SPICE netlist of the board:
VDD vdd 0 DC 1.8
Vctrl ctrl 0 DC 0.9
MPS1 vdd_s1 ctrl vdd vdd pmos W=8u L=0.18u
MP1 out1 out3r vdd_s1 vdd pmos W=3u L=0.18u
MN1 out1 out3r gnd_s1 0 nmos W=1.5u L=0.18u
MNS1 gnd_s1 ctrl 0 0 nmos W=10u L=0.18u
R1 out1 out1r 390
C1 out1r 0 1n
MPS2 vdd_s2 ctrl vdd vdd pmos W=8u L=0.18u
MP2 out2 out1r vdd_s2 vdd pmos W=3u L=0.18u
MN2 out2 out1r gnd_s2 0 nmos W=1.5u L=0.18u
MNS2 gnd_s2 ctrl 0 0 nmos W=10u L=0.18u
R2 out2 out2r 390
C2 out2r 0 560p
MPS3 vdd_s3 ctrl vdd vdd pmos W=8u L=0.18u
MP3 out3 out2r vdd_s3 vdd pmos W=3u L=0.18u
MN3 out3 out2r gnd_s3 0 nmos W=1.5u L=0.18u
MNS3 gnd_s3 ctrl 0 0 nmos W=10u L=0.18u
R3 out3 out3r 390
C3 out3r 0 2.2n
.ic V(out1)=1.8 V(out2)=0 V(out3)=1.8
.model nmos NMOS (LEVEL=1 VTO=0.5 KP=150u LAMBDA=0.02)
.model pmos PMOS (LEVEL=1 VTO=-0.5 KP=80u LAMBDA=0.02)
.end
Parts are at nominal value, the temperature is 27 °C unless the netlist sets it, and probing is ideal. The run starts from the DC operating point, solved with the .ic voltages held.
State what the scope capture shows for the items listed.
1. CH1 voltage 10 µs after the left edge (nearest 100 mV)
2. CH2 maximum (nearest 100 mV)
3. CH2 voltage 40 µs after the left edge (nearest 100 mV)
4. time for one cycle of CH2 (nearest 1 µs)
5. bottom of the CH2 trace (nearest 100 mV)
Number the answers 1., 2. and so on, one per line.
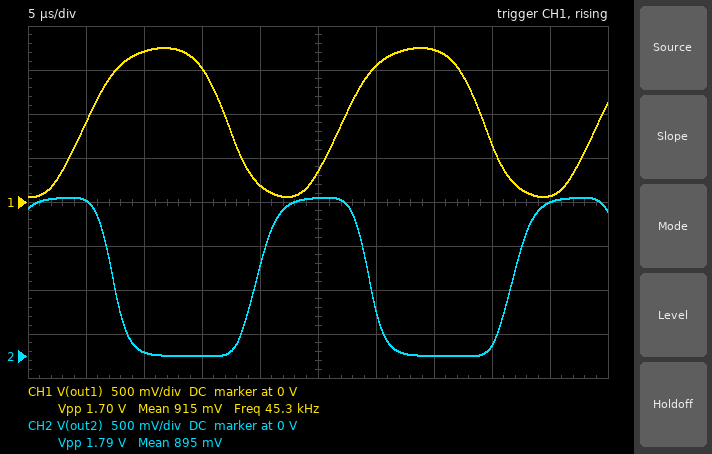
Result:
1. 1.7 V
2. 1.8 V
3. 100 mV
4. 22 µs
5. 0 V
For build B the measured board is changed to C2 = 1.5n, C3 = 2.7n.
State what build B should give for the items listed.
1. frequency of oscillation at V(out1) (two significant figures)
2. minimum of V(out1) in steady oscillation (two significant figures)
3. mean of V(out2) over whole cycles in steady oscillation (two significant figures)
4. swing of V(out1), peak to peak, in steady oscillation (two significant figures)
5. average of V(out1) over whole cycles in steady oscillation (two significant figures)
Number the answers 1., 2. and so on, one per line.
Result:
1. 32 kHz
2. 3.2 mV
3. 790 mV
4. 1.8 V
5. 910 mV
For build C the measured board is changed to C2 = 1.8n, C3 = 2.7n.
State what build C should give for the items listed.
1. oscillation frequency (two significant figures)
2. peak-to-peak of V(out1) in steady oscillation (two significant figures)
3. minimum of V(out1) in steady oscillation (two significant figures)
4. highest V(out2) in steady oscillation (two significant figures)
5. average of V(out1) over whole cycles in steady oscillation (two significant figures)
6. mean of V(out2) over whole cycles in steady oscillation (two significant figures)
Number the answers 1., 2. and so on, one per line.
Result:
1. 30 kHz
2. 1.8 V
3. 1.3 mV
4. 1.7 V
5. 890 mV
6. 800 mV
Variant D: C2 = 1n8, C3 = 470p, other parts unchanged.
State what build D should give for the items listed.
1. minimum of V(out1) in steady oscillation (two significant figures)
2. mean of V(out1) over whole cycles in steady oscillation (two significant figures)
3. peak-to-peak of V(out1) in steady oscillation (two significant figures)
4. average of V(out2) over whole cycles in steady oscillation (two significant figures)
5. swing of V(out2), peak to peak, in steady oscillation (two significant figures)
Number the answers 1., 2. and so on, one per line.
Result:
1. 7.0 mV
2. 780 mV
3. 1.7 V
4. 890 mV
5. 1.4 V
